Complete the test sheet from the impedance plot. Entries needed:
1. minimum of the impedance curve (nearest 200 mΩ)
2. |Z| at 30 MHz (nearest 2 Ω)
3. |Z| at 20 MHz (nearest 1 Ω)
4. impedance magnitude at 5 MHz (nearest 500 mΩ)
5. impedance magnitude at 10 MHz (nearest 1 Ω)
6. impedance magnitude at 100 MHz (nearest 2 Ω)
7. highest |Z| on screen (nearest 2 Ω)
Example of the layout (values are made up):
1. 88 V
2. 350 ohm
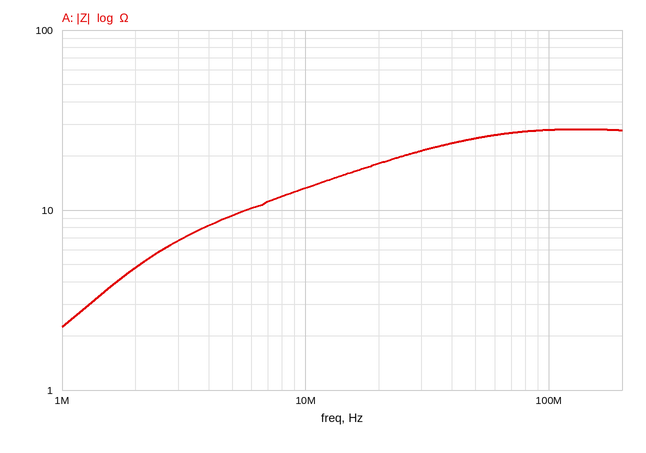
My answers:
1. 2.2 Ω
2. 22 Ω
3. 18 Ω
4. 9.5 Ω
5. 13 Ω
6. 28 Ω
7. 28 Ω
